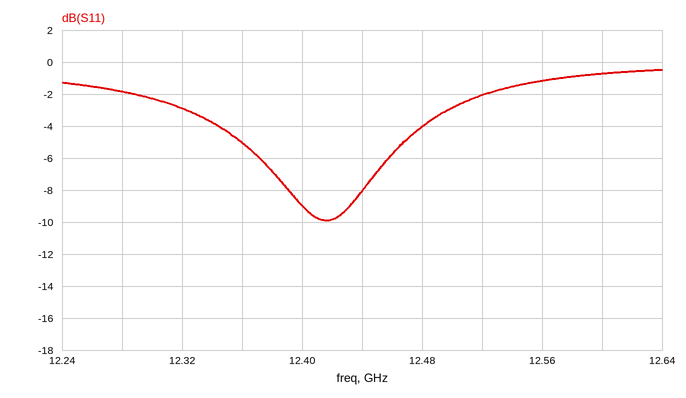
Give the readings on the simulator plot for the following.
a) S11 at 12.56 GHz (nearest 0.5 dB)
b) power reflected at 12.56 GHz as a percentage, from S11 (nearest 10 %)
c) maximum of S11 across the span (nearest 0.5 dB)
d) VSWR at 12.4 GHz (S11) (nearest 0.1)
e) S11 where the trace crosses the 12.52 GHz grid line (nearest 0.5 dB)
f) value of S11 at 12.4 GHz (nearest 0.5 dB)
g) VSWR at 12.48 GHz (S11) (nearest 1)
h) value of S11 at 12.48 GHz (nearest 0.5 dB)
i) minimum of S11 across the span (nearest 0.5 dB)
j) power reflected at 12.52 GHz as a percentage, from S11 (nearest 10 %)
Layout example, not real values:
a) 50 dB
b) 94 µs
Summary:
a) -1.0 dB
b) 80 %
c) -0.5 dB
d) 2.1
e) -2.0 dB
f) -9.0 dB
g) 4
h) -4.0 dB
i) -10.0 dB
j) 60 %
